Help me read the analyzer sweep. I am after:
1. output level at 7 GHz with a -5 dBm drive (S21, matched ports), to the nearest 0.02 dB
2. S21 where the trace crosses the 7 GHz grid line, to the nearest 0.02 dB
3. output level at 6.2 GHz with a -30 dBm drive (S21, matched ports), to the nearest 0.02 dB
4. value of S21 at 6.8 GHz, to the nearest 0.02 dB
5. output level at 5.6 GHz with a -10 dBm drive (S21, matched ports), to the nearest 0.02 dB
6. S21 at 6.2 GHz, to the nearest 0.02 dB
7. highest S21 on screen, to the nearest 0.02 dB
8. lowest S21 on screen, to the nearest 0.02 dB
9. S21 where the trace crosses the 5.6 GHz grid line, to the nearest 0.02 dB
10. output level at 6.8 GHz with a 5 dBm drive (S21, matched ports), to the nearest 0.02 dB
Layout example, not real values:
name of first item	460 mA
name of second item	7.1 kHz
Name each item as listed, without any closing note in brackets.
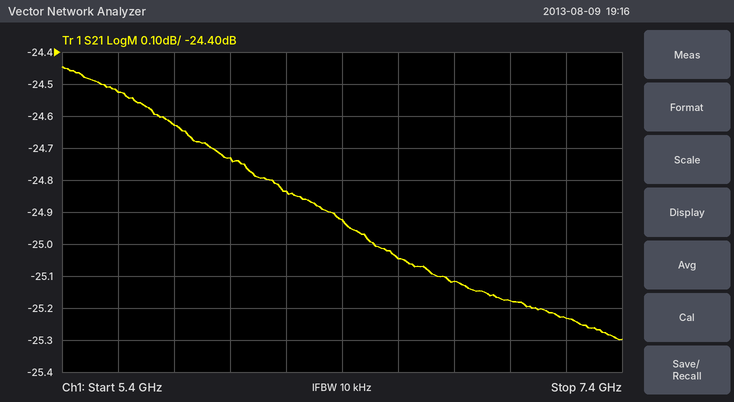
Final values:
output level at 7 GHz with a -5 dBm drive (S21, matched ports), to the nearest 0.02 dB	-30.18 dBm
S21 where the trace crosses the 7 GHz grid line, to the nearest 0.02 dB	-25.18 dB
output level at 6.2 GHz with a -30 dBm drive (S21, matched ports), to the nearest 0.02 dB	-54.84 dBm
value of S21 at 6.8 GHz, to the nearest 0.02 dB	-25.12 dB
output level at 5.6 GHz with a -10 dBm drive (S21, matched ports), to the nearest 0.02 dB	-34.52 dBm
S21 at 6.2 GHz, to the nearest 0.02 dB	-24.84 dB
highest S21 on screen, to the nearest 0.02 dB	-24.44 dB
lowest S21 on screen, to the nearest 0.02 dB	-25.30 dB
S21 where the trace crosses the 5.6 GHz grid line, to the nearest 0.02 dB	-24.52 dB
output level at 6.8 GHz with a 5 dBm drive (S21, matched ports), to the nearest 0.02 dB	-20.12 dBm
